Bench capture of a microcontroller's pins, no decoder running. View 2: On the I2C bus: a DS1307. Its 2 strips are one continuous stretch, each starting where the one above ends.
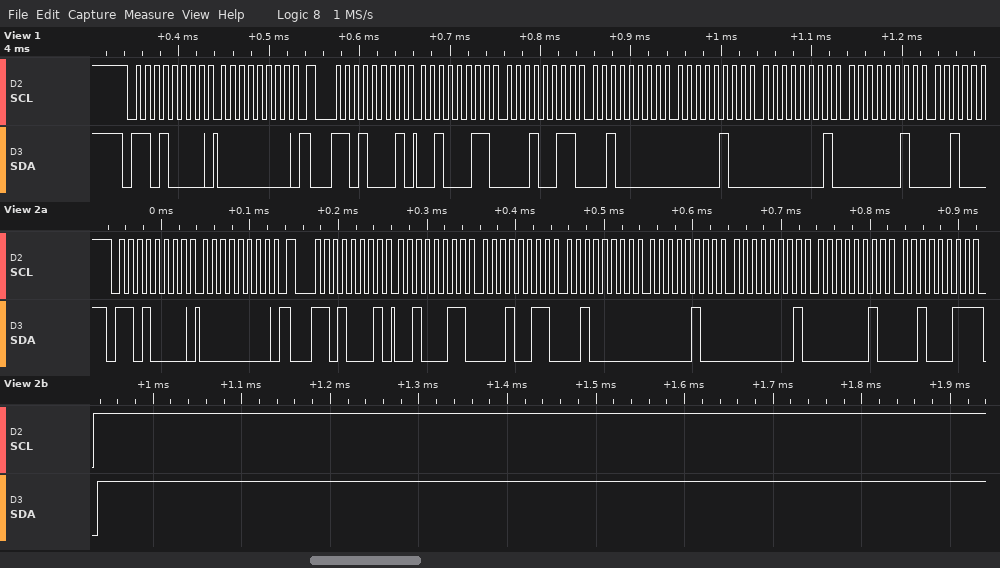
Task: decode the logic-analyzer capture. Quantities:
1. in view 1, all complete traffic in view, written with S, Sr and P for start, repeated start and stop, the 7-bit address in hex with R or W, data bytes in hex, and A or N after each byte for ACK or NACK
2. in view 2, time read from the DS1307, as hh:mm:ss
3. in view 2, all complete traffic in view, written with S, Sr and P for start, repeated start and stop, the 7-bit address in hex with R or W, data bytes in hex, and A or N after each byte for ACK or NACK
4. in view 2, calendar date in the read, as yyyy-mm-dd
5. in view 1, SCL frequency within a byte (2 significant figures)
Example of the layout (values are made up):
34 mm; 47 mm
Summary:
S 68W A 00 A Sr 68R A 23 A 13 A 20 A 04 A 01 A 02 A; 20:13:23; S 68W A 00 A Sr 68R A 23 A 13 A 20 A 04 A 01 A 02 A 23 N P; 2023-02-01; 100 kHz
